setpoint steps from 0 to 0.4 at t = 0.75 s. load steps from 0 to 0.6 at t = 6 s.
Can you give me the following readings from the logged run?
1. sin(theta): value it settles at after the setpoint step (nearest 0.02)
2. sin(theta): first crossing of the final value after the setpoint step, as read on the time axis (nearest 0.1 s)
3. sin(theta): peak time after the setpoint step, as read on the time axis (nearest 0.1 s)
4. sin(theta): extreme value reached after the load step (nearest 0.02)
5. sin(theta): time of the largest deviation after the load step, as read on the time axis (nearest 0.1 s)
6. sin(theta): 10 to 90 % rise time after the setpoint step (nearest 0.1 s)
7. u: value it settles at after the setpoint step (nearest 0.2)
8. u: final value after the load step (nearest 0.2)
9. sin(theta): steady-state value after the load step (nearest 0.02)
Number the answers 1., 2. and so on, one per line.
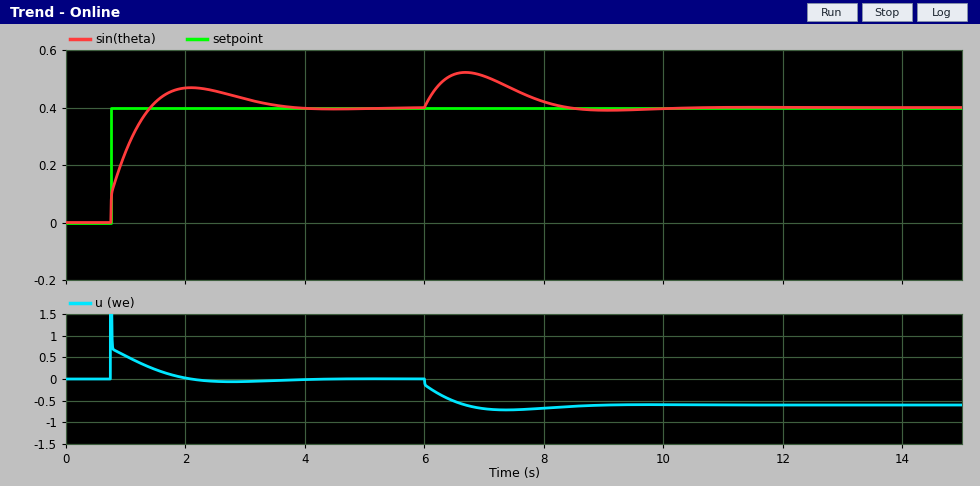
1. 0.40
2. 1.4 s
3. 2.1 s
4. 0.52
5. 6.7 s
6. 0.5 s
7. 0.0
8. -0.6
9. 0.40
